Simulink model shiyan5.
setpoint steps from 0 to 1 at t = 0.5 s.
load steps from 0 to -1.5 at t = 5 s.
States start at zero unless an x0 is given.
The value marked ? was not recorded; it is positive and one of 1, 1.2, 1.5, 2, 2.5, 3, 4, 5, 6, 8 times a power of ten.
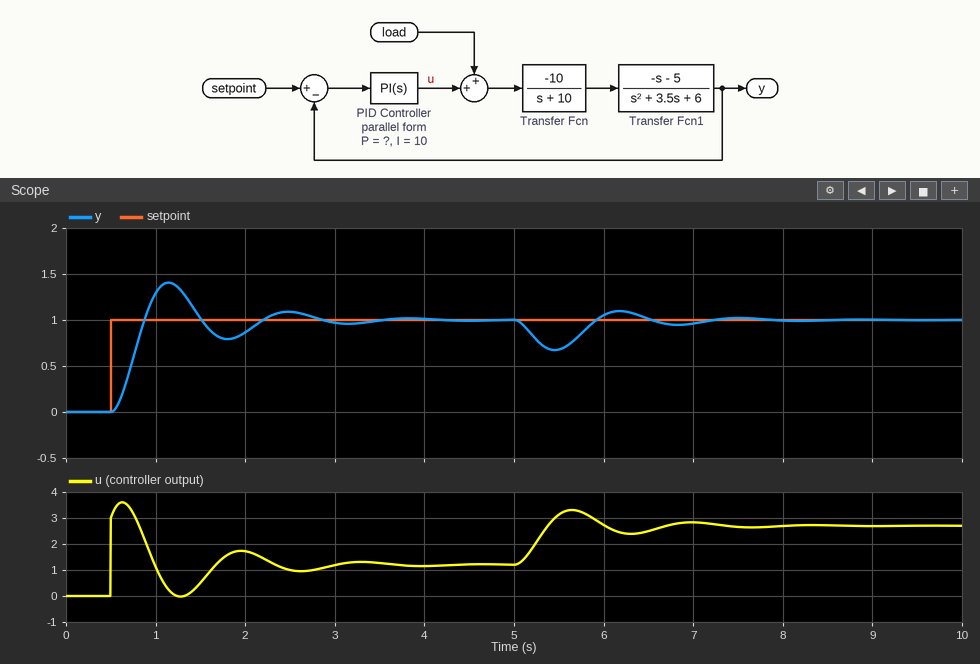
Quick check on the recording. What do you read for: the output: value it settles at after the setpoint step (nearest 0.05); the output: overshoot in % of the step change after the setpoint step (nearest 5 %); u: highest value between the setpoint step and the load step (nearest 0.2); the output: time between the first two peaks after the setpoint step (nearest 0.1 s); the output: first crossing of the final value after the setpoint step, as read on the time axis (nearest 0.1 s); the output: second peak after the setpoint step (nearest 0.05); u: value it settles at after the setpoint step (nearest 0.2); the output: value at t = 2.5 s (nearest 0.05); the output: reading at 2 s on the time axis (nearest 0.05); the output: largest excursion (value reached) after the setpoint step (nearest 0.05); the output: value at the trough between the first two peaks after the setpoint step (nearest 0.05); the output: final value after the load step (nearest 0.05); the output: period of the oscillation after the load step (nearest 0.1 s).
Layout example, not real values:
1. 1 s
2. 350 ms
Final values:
1. 1.00
2. 40 %
3. 3.6
4. 1.3 s
5. 0.9 s
6. 1.10
7. 1.2
8. 1.10
9. 0.85
10. 1.40
11. 0.80
12. 1.00
13. 1.4 s
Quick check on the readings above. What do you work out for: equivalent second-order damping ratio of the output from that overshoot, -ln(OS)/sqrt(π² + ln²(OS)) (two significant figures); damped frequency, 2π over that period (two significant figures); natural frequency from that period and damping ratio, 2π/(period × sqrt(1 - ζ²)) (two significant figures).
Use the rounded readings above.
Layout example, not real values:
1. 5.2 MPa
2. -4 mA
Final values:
1. 0.28
2. 4.8 rad/s
3. 5.0 rad/s
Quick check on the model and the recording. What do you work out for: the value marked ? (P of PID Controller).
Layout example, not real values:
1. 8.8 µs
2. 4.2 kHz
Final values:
1. 3
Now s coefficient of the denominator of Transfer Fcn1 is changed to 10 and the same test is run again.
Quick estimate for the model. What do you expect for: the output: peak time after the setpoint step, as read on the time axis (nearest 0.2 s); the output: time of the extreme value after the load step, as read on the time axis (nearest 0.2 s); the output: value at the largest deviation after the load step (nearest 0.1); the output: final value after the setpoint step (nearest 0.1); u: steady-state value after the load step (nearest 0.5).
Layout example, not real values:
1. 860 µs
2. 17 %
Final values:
1. 1.6 s
2. 5.6 s
3. 0.8
4. 1.0
5. 2.5
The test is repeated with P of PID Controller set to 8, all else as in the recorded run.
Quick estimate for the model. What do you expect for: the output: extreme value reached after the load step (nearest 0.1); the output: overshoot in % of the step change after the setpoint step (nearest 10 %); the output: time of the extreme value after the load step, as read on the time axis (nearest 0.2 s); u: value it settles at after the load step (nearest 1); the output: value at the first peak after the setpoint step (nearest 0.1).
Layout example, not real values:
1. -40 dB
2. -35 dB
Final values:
1. 0.8
2. 30 %
3. 5.4 s
4. 3
5. 1.3
